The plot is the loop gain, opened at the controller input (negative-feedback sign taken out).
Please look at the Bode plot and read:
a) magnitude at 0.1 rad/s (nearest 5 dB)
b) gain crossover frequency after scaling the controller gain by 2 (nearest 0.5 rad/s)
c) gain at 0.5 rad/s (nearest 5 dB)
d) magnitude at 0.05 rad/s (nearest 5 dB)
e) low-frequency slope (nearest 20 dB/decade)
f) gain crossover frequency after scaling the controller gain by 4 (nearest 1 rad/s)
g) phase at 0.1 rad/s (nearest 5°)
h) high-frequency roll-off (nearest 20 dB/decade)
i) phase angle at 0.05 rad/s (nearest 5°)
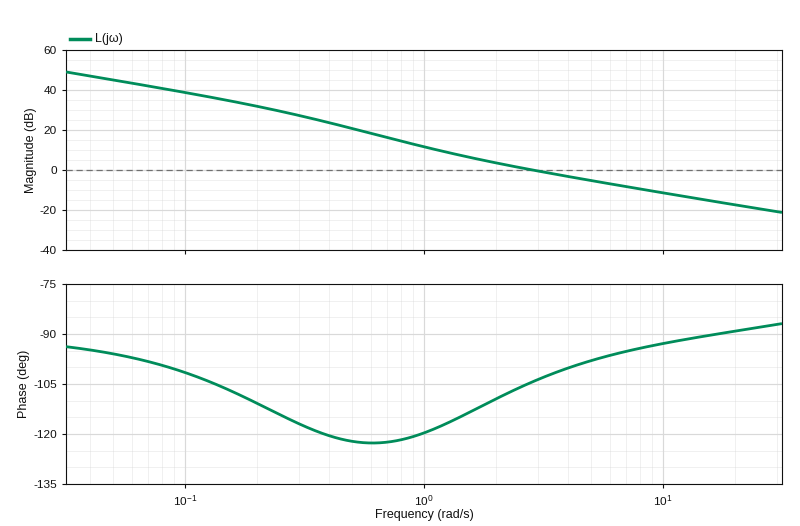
40 dB
5.5 rad/s
20 dB
45 dB
-20 dB/decade
11 rad/s
-100°
-20 dB/decade
-95°
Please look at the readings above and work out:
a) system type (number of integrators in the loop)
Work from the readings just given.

1
